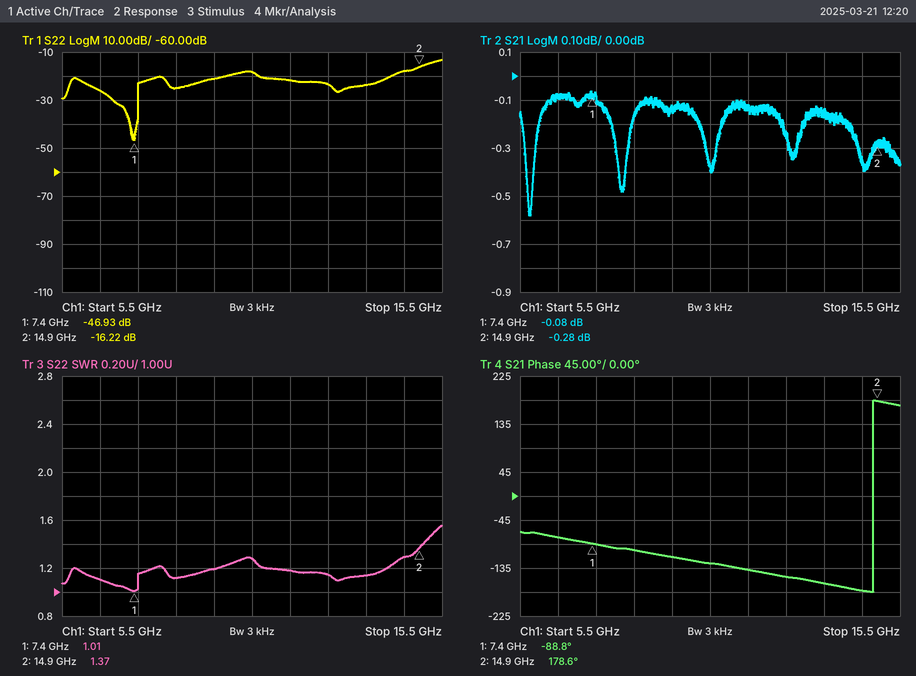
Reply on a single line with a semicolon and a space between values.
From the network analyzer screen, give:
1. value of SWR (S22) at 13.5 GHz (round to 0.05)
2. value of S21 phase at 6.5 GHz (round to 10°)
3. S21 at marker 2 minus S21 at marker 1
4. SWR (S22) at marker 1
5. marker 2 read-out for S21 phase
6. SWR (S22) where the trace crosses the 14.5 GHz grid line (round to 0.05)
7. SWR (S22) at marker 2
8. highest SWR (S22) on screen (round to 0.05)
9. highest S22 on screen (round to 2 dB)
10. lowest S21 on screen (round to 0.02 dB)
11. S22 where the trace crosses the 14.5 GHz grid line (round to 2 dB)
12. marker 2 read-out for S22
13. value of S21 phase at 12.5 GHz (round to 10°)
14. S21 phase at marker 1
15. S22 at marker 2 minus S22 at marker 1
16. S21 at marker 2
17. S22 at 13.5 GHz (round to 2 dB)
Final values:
1.15; -80°; -0.20 dB; 1.01; 178.6°; 1.30; 1.37; 1.55; -14 dB; -0.58 dB; -18 dB; -16.22 dB; -150°; -88.8°; 30.71 dB; -0.28 dB; -24 dB
